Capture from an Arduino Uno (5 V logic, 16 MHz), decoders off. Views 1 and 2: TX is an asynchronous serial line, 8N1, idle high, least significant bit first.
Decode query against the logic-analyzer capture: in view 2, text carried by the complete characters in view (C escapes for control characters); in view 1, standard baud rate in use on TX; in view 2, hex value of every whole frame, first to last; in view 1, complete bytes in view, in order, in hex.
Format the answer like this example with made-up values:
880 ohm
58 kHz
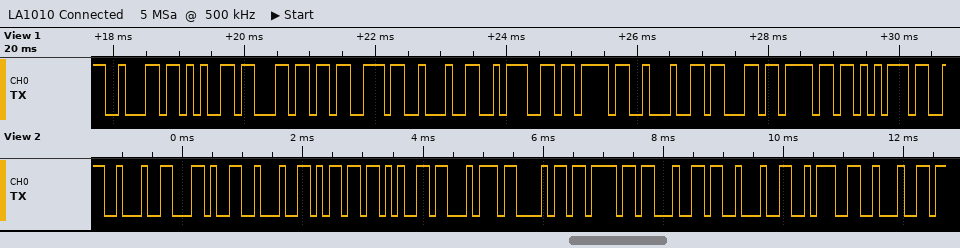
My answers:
"\",\"method\":\""
9600 baud
22 2C 22 6D 65 74 68 6F 64 22 3A 22
62 65 6C 73 22 3A 7B 22 63 6F 75
